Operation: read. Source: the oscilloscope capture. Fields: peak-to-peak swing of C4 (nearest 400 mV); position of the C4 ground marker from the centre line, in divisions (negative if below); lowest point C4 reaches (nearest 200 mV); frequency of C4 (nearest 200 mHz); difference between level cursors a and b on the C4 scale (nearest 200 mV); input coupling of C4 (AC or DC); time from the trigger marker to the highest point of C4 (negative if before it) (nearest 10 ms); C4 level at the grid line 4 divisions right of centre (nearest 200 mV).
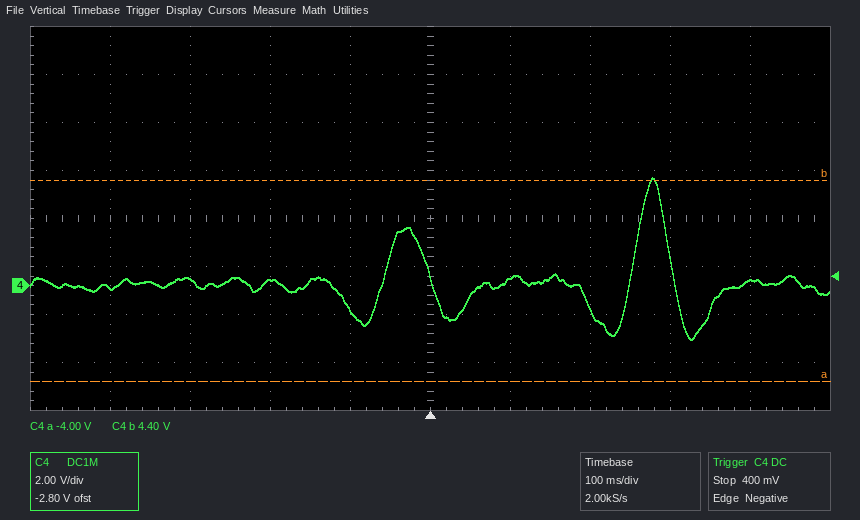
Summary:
6.8 V
-1.4 div
-2.2 V
3.2 Hz
8.4 V
DC
+280 ms
200 mV
